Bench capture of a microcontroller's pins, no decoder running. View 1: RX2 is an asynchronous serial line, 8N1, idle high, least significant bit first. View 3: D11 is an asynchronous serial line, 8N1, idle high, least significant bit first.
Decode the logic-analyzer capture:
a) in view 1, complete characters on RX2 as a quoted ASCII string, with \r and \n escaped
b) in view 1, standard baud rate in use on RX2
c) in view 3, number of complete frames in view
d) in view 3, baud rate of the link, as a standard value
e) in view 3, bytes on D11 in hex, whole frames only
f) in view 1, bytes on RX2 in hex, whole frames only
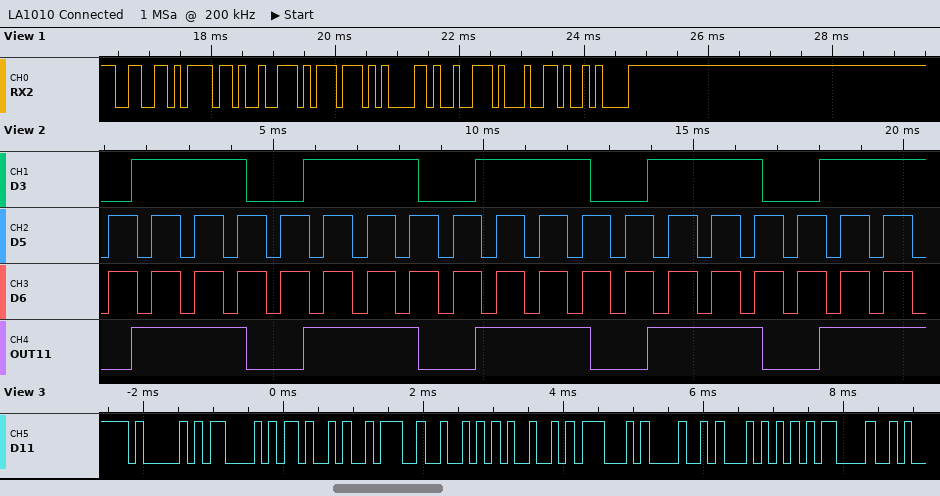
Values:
"forward\n"
9600 baud
10
9600 baud
41 43 4B 3A 52 49 47 48 54 0D
66 6F 72 77 61 72 64 0A
